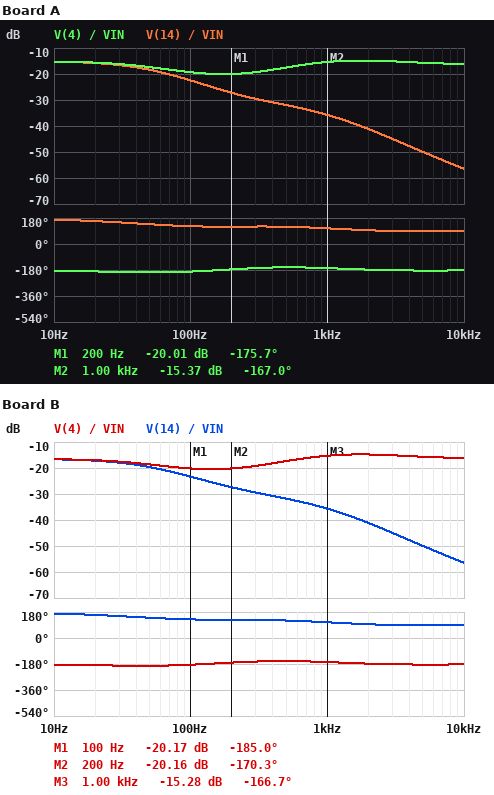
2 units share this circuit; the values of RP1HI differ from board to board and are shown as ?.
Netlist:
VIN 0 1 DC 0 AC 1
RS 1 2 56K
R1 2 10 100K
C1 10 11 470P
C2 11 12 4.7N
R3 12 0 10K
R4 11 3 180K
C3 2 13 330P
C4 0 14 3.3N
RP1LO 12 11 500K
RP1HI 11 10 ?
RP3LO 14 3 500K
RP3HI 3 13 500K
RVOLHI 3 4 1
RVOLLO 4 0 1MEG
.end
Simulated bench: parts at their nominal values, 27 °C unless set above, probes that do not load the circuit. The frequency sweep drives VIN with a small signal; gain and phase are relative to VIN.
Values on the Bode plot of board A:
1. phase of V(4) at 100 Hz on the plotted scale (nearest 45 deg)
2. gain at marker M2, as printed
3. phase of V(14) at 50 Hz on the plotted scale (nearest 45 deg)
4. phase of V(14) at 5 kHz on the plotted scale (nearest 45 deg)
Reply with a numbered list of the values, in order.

1. -180 deg
2. -15.37 dB
3. 135 deg
4. 90 deg
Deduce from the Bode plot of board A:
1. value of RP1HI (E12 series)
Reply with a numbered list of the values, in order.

1. 1.2 MΩ
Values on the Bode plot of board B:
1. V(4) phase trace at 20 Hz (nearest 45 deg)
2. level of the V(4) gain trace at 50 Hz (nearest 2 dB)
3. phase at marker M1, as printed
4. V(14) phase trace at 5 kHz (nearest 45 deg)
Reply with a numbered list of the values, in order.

1. -180 deg
2. -18 dB
3. -185.0 deg
4. 90 deg
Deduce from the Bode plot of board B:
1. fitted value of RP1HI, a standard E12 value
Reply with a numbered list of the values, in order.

1. 1.5 MΩ
